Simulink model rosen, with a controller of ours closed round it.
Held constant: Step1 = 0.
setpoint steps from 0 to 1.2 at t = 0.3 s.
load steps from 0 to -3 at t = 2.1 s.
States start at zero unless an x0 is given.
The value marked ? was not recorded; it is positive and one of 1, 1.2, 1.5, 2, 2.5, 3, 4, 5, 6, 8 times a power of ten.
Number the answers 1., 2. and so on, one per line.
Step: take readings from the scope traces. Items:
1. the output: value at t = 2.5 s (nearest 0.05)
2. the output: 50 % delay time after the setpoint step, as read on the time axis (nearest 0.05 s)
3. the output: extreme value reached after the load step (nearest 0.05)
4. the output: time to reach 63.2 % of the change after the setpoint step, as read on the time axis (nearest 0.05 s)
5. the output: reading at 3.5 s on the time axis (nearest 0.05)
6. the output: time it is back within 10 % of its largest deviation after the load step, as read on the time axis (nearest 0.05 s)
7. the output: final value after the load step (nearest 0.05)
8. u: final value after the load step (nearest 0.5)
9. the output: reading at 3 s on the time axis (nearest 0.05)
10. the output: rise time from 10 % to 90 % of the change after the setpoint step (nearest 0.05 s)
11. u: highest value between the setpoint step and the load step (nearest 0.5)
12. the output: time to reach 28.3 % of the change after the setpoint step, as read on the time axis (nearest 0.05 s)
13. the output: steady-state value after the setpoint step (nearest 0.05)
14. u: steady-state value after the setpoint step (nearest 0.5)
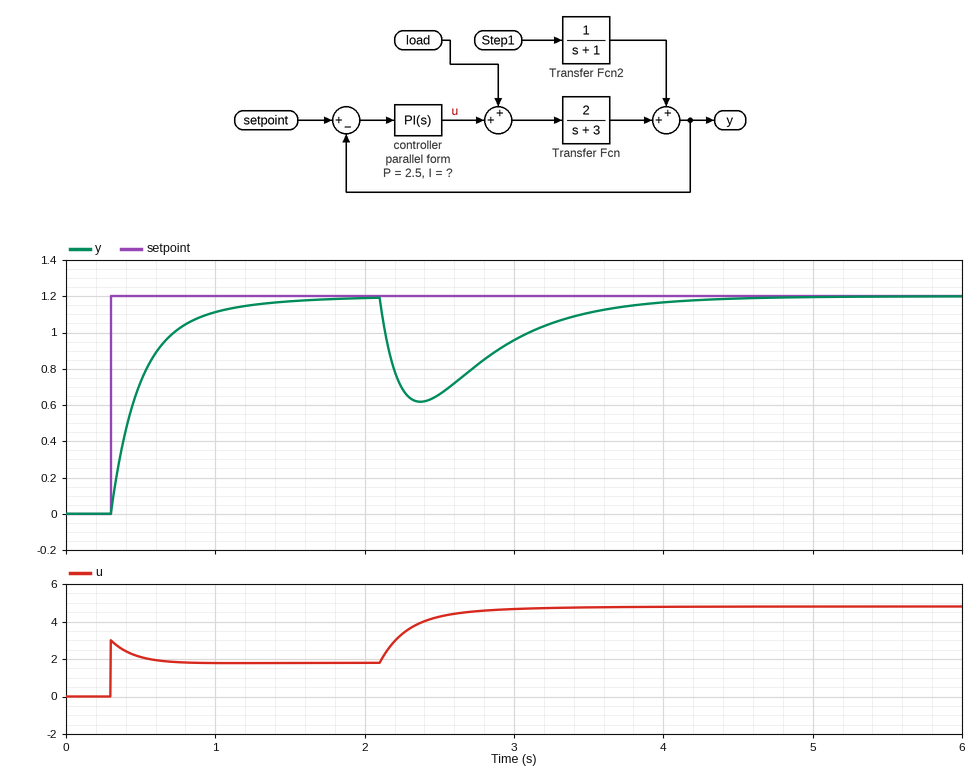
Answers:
1. 0.65
2. 0.45 s
3. 0.60
4. 0.50 s
5. 1.10
6. 3.75 s
7. 1.20
8. 5.0
9. 0.95
10. 0.55 s
11. 3.0
12. 0.35 s
13. 1.20
14. 2.0
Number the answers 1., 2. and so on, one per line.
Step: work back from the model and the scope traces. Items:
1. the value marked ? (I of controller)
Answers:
1. 6
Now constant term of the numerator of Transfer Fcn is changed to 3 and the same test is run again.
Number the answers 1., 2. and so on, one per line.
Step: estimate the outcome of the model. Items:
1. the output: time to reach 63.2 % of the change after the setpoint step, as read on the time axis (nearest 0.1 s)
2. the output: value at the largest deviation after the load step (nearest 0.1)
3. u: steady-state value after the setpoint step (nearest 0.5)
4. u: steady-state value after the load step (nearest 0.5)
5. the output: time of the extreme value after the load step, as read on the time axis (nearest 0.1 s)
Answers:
1. 0.4 s
2. 0.5
3. 1.0
4. 4.0
5. 2.3 s
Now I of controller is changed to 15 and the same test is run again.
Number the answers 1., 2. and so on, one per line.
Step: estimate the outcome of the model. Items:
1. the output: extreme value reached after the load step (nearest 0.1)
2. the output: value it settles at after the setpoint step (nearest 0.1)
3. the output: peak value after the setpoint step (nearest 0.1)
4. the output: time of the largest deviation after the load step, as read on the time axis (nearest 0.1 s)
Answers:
1. 0.7
2. 1.2
3. 1.3
4. 2.3 s
